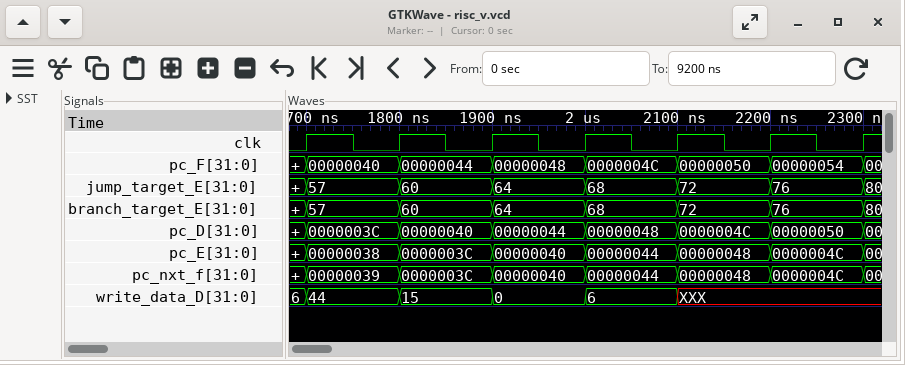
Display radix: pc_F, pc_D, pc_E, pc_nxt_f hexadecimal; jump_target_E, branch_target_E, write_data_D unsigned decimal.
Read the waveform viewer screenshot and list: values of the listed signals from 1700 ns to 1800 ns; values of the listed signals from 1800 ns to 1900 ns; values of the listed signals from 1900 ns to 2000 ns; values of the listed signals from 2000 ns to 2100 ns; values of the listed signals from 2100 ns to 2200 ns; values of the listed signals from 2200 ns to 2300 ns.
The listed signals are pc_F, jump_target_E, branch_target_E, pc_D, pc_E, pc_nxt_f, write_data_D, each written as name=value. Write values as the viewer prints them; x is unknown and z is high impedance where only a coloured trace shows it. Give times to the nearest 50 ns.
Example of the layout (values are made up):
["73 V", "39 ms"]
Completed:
["pc_F=00000040, jump_target_E=57, branch_target_E=57, pc_D=0000003C, pc_E=00000038, pc_nxt_f=00000039, write_data_D=44", "pc_F=00000044, jump_target_E=60, branch_target_E=60, pc_D=00000040, pc_E=0000003C, pc_nxt_f=0000003C, write_data_D=15", "pc_F=00000048, jump_target_E=64, branch_target_E=64, pc_D=00000044, pc_E=00000040, pc_nxt_f=00000040, write_data_D=0", "pc_F=0000004C, jump_target_E=68, branch_target_E=68, pc_D=00000048, pc_E=00000044, pc_nxt_f=00000044, write_data_D=6", "pc_F=00000050, jump_target_E=72, branch_target_E=72, pc_D=0000004C, pc_E=00000048, pc_nxt_f=00000048, write_data_D=XXX", "pc_F=00000054, jump_target_E=76, branch_target_E=76, pc_D=00000050, pc_E=0000004C, pc_nxt_f=0000004C, write_data_D=XXX"]
